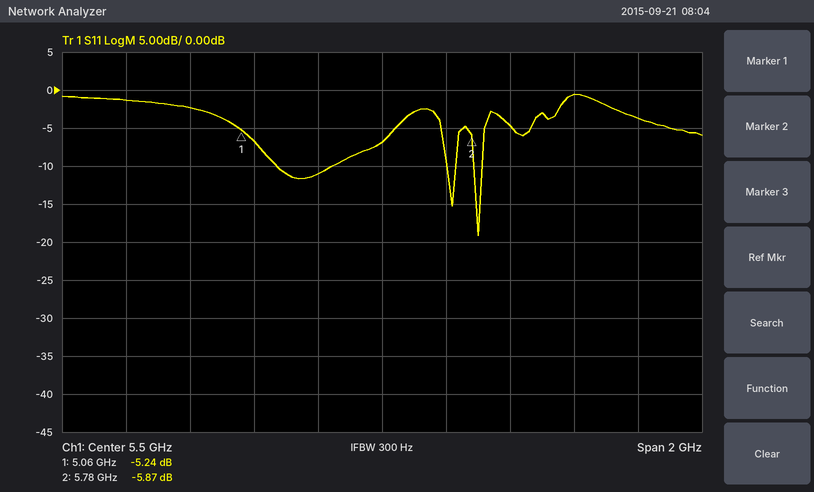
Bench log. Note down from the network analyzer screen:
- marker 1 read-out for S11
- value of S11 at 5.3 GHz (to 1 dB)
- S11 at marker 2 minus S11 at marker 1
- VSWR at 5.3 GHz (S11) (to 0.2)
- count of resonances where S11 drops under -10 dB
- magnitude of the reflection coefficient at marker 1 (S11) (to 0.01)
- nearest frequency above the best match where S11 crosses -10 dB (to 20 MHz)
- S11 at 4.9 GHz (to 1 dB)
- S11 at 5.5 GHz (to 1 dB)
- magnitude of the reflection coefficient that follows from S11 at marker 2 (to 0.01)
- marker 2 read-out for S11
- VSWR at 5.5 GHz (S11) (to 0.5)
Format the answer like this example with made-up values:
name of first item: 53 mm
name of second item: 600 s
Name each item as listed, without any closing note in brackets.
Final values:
marker 1 read-out for S11: -5.24 dB
value of S11 at 5.3 GHz: -11 dB
S11 at marker 2 minus S11 at marker 1: -0.63 dB
VSWR at 5.3 GHz (S11): 1.8
count of resonances where S11 drops under -10 dB: 3
magnitude of the reflection coefficient at marker 1 (S11): 0.55
nearest frequency above the best match where S11 crosses -10 dB: 5.82 GHz
S11 at 4.9 GHz: -2 dB
S11 at 5.5 GHz: -7 dB
magnitude of the reflection coefficient that follows from S11 at marker 2: 0.51
marker 2 read-out for S11: -5.87 dB
VSWR at 5.5 GHz (S11): 2.5
